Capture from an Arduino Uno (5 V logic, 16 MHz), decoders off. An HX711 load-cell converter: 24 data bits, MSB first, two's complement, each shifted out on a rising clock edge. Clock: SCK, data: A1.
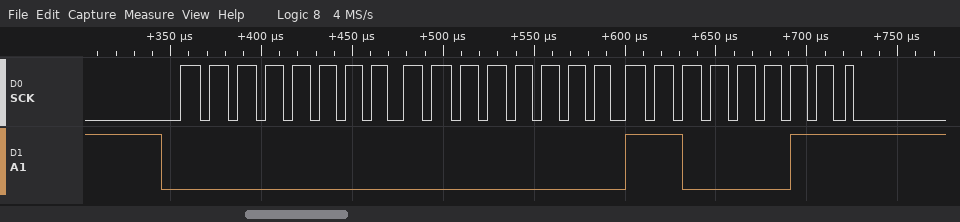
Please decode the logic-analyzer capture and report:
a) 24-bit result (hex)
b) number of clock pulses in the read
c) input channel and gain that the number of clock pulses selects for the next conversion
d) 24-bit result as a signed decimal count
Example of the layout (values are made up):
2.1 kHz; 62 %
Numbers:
0x0000C3; 25; channel A, gain 128; 195
